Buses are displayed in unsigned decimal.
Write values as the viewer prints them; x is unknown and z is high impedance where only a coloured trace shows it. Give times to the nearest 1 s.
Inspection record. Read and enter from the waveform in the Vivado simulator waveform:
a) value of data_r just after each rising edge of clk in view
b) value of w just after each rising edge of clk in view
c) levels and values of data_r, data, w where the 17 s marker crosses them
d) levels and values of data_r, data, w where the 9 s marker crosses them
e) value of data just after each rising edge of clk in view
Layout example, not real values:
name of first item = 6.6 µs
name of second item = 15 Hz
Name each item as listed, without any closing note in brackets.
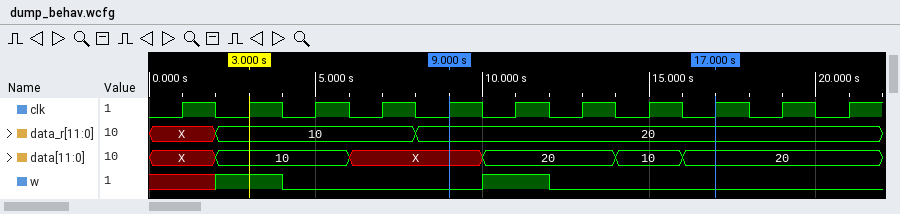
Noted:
value of data_r just after each rising edge of clk in view = X, 10, 10, 10, 20, 20, 20, 20, 20, 20, 20
value of w just after each rising edge of clk in view = x 1 0 0 0 1 0 0 0 0 0
levels and values of data_r, data, w where the 17 s marker crosses them = data_r=20, data=20, w=0
levels and values of data_r, data, w where the 9 s marker crosses them = data_r=20, data=X, w=0
value of data just after each rising edge of clk in view = X, 10, 10, X, X, 20, 20, 10, 20, 20, 20
